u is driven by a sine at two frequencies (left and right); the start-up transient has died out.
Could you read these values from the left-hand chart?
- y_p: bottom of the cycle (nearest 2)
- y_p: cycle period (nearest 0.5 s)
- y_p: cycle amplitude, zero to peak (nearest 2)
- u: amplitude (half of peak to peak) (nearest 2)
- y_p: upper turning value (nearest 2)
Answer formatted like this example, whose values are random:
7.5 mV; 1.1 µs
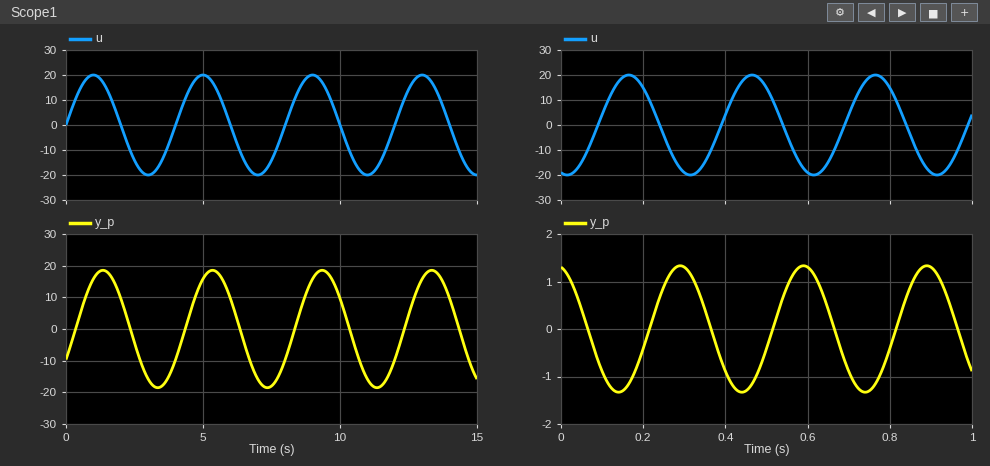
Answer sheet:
-18; 4.0 s; 18; 20; 18
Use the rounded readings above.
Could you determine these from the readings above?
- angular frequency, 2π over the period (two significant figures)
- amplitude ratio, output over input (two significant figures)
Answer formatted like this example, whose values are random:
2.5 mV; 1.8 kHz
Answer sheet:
1.6 rad/s; 0.90
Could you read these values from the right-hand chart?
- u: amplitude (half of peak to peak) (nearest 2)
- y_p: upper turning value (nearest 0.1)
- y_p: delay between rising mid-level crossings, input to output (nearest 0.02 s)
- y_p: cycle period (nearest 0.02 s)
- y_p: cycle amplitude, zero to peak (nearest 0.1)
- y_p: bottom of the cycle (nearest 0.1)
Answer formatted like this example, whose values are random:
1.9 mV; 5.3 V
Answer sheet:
20; 1.3; 0.12 s; 0.30 s; 1.3; -1.3
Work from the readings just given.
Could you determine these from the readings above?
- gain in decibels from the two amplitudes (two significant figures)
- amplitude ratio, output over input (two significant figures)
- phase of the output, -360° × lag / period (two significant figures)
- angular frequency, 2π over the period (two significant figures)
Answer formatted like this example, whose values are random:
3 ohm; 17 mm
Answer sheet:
-24 dB; 0.065; -140°; 21 rad/s
